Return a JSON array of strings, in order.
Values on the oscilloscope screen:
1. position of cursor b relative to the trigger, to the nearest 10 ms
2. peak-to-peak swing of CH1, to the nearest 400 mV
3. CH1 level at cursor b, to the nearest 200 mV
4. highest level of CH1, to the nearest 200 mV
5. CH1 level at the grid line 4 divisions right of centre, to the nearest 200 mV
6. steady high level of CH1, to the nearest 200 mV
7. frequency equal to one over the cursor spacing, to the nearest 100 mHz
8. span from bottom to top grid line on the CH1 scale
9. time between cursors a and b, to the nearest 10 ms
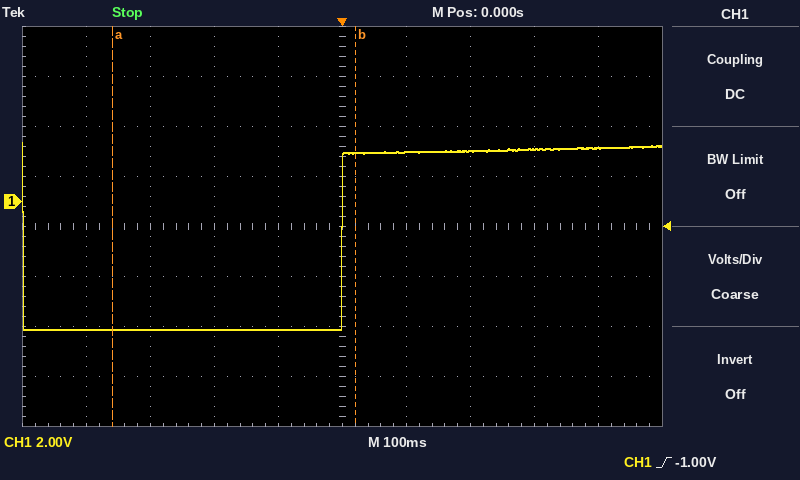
["+20 ms", "7.6 V", "2.0 V", "2.4 V", "2.2 V", "2.0 V", "2.6 Hz", "16 V", "380 ms"]
